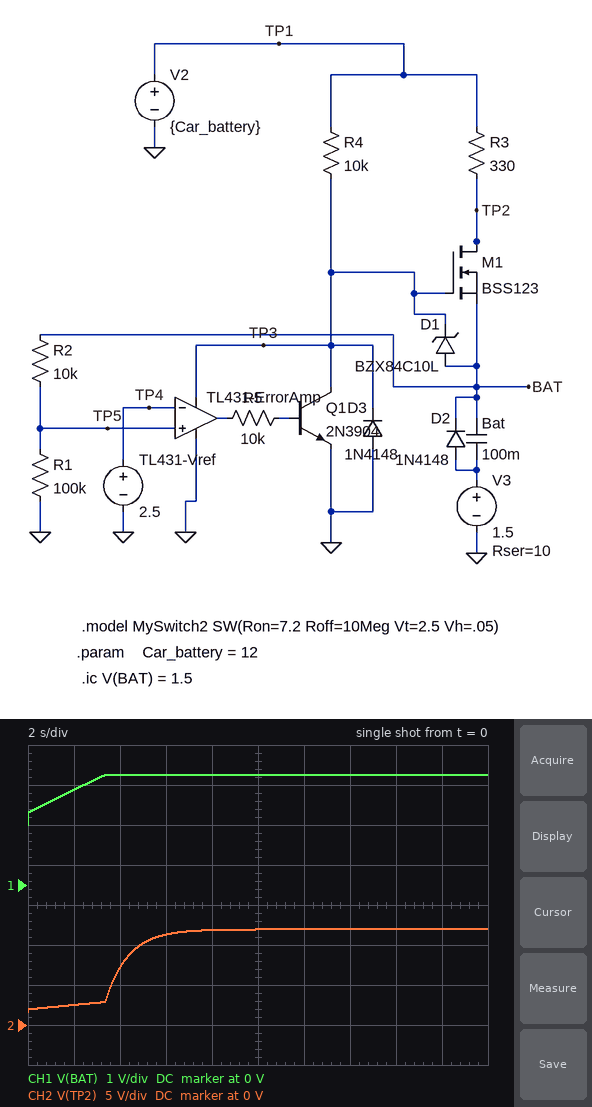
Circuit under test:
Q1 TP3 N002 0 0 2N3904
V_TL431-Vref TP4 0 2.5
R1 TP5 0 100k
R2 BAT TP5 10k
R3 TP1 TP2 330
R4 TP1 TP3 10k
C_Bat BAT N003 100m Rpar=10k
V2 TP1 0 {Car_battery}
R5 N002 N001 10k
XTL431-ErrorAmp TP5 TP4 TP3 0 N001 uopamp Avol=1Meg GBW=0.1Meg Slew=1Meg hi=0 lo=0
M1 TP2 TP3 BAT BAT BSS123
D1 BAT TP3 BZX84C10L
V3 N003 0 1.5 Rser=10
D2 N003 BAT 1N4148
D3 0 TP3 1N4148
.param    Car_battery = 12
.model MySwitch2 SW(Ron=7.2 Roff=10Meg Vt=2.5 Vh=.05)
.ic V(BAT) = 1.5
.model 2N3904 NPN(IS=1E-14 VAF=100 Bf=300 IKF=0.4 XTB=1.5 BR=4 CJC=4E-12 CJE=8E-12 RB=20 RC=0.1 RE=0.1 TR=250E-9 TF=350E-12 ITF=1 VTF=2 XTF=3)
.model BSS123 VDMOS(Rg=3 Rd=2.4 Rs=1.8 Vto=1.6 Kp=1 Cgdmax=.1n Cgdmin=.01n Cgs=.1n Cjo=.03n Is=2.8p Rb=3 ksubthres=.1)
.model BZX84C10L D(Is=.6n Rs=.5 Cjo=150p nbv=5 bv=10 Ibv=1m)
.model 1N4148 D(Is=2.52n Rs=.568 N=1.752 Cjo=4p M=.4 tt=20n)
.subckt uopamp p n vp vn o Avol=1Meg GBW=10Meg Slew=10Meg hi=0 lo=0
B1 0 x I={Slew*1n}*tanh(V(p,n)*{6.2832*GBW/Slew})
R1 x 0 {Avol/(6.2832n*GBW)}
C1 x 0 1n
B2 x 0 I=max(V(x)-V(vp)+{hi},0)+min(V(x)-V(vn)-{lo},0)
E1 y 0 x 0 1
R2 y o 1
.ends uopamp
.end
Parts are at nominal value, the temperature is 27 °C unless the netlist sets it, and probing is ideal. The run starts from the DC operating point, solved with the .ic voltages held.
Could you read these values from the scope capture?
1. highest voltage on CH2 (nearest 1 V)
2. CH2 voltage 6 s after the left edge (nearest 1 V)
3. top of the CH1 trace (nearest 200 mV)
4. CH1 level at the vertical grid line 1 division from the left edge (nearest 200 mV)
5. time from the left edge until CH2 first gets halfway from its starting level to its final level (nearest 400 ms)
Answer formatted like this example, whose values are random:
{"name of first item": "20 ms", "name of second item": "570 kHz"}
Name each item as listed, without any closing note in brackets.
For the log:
{"highest voltage on CH2": "12 V", "CH2 voltage 6 s after the left edge": "11 V", "top of the CH1 trace": "2.8 V", "CH1 level at the vertical grid line 1 division from the left edge": "2.4 V", "time from the left edge until CH2 first gets halfway from its starting level to its final level": "4.0 s"}
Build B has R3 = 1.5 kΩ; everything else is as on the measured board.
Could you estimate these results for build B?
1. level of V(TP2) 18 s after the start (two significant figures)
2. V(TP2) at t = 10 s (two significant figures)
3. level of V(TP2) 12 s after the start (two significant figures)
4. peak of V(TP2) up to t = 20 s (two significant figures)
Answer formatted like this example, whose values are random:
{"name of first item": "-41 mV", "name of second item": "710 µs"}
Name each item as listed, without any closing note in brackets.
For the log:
{"level of V(TP2) 18 s after the start": "2.8 V", "V(TP2) at t = 10 s": "2.3 V", "level of V(TP2) 12 s after the start": "2.4 V", "peak of V(TP2) up to t = 20 s": "10 V"}
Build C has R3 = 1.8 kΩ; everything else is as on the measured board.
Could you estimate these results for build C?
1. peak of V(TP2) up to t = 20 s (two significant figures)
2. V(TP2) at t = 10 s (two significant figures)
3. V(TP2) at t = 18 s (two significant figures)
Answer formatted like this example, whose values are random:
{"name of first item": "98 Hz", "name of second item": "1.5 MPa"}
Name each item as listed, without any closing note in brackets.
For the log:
{"peak of V(TP2) up to t = 20 s": "2.7 V", "V(TP2) at t = 10 s": "2.1 V", "V(TP2) at t = 18 s": "2.6 V"}
